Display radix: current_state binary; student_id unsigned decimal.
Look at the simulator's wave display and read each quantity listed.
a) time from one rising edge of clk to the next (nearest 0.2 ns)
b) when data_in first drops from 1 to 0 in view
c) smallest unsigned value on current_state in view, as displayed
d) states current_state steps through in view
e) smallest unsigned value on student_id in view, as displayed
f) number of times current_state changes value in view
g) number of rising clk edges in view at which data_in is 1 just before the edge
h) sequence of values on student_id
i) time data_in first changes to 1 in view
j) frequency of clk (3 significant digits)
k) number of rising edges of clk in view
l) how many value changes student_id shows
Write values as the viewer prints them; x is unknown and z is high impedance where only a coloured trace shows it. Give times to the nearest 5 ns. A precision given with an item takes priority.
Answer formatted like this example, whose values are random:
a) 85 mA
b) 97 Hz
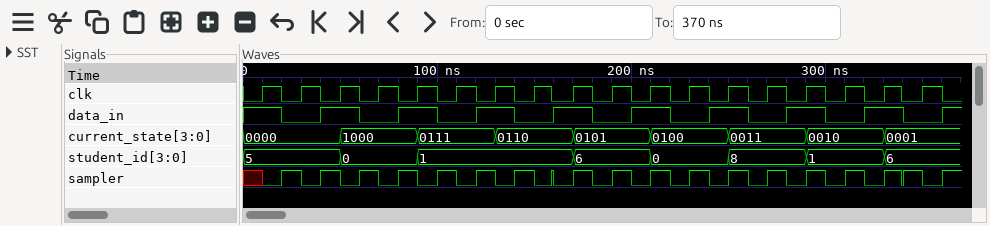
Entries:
a) 20 ns
b) 20 ns
c) 0000
d) 0000, 1000, 0111, 0110, 0101, 0100, 0011, 0010, 0001
e) 0
f) 8
g) 9
h) 5, 0, 1, 6, 0, 8, 1, 6
i) 40 ns
j) 50.0 MHz
k) 18
l) 7
